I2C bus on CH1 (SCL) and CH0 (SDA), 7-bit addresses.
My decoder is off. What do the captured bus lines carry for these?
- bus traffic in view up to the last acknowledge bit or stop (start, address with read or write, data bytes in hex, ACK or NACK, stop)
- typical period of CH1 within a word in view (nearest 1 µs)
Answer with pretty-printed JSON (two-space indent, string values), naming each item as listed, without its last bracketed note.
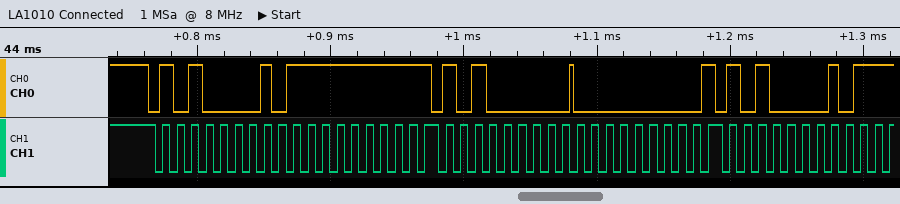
{
  "bus traffic in view up to the last acknowledge bit or stop": "start, address 50 read ACK, FF NACK, repeated start, address 50 write ACK, 00 ACK, repeated start, address 50 read ACK",
  "typical period of CH1 within a word in view": "11 µs"
}
